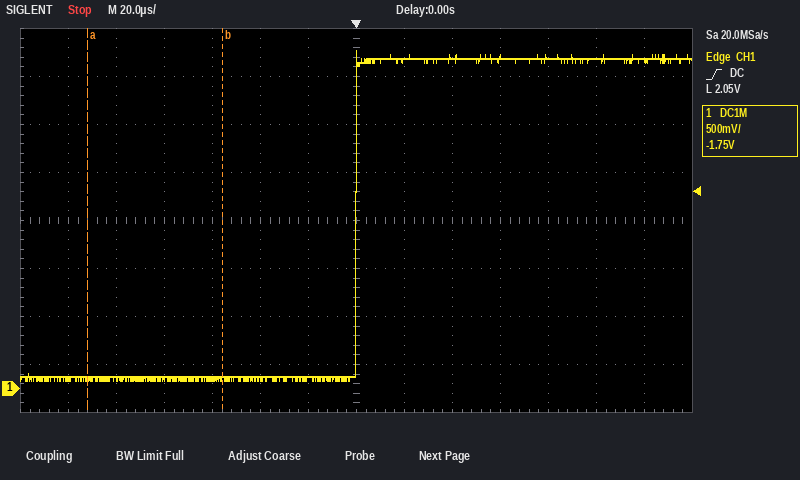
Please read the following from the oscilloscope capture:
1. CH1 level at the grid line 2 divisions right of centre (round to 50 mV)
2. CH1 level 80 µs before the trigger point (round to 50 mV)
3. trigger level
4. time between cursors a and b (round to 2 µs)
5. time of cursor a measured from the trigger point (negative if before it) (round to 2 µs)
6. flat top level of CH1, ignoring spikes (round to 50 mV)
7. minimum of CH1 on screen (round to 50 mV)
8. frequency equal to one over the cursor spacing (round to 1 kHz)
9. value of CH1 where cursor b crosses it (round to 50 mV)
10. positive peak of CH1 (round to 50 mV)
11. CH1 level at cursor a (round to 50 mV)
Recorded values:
3.45 V
100 mV
2.05 V
56 µs
-112 µs
3.45 V
100 mV
18 kHz
100 mV
3.50 V
100 mV
